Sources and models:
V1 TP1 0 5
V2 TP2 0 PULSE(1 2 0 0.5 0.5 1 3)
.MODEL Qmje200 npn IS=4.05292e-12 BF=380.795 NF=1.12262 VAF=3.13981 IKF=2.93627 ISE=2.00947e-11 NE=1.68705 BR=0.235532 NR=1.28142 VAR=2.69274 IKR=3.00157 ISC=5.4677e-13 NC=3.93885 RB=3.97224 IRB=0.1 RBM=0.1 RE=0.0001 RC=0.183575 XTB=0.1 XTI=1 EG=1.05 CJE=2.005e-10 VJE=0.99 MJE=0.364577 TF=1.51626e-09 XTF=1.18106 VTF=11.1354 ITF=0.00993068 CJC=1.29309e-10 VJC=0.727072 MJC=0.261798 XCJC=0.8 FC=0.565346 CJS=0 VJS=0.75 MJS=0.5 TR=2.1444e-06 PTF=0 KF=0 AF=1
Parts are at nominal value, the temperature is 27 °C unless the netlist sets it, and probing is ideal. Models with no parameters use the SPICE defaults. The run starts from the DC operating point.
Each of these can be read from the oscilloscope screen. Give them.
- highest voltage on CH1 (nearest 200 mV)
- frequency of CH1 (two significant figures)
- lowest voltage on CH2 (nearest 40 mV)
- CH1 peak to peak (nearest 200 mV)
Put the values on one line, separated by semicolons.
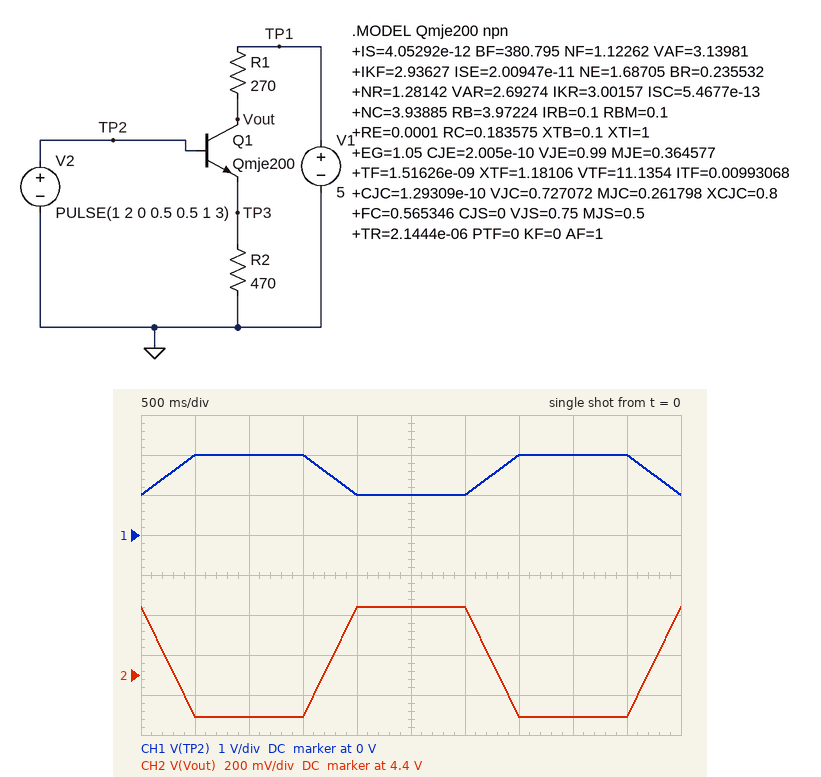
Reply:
2.0 V; 330 mHz; 4.20 V; 1.0 V
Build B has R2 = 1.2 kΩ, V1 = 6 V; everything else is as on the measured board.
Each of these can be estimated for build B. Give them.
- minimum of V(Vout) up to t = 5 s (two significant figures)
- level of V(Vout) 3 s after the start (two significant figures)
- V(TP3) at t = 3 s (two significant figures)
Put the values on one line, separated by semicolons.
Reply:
5.7 V; 5.9 V; 490 mV
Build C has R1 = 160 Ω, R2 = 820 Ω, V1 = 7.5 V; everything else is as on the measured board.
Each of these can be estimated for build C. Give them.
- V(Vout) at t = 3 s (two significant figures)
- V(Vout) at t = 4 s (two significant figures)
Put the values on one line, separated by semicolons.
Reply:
7.4 V; 7.2 V
